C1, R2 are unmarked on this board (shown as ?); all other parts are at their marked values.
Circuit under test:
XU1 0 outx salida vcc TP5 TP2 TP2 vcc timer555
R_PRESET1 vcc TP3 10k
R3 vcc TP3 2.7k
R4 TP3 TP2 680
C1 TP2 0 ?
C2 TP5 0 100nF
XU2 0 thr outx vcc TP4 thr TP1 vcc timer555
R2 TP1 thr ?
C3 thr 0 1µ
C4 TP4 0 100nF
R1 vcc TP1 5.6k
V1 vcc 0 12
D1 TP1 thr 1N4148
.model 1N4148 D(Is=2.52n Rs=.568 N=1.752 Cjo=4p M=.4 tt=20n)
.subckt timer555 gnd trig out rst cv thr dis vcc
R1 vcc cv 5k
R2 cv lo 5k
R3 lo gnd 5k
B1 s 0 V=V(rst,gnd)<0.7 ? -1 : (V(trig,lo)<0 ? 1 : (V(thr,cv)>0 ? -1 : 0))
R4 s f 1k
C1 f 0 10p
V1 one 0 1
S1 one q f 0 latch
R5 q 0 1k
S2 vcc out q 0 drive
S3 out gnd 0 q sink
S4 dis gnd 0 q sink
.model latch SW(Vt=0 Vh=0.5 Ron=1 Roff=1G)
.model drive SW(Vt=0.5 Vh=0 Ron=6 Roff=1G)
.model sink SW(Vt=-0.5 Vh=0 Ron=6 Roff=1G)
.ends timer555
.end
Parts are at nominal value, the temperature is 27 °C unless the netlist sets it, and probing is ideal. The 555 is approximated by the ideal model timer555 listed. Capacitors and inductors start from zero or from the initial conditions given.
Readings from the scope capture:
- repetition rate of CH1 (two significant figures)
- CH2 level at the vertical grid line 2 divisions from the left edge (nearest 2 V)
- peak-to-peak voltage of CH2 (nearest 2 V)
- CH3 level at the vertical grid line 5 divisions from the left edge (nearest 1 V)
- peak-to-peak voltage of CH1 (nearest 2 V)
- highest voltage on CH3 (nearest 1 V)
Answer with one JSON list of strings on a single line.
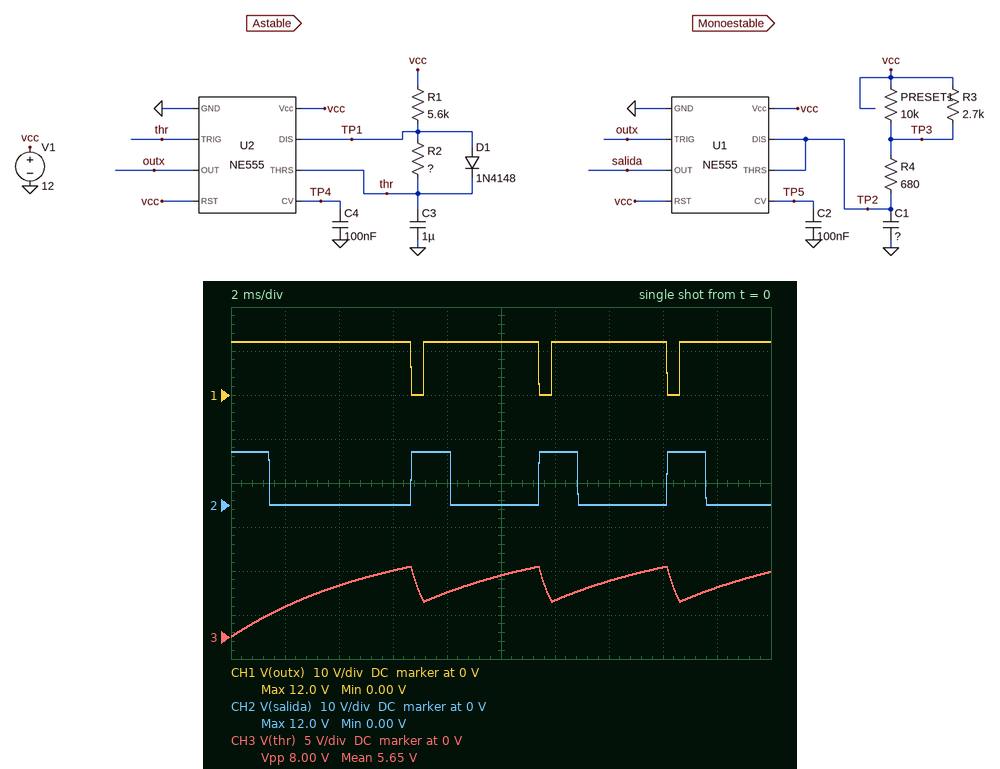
["210 Hz", "0 V", "12 V", "7 V", "12 V", "8 V"]
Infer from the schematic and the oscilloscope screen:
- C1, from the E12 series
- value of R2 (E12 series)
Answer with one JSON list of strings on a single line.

["470 nF", "680 Ω"]
